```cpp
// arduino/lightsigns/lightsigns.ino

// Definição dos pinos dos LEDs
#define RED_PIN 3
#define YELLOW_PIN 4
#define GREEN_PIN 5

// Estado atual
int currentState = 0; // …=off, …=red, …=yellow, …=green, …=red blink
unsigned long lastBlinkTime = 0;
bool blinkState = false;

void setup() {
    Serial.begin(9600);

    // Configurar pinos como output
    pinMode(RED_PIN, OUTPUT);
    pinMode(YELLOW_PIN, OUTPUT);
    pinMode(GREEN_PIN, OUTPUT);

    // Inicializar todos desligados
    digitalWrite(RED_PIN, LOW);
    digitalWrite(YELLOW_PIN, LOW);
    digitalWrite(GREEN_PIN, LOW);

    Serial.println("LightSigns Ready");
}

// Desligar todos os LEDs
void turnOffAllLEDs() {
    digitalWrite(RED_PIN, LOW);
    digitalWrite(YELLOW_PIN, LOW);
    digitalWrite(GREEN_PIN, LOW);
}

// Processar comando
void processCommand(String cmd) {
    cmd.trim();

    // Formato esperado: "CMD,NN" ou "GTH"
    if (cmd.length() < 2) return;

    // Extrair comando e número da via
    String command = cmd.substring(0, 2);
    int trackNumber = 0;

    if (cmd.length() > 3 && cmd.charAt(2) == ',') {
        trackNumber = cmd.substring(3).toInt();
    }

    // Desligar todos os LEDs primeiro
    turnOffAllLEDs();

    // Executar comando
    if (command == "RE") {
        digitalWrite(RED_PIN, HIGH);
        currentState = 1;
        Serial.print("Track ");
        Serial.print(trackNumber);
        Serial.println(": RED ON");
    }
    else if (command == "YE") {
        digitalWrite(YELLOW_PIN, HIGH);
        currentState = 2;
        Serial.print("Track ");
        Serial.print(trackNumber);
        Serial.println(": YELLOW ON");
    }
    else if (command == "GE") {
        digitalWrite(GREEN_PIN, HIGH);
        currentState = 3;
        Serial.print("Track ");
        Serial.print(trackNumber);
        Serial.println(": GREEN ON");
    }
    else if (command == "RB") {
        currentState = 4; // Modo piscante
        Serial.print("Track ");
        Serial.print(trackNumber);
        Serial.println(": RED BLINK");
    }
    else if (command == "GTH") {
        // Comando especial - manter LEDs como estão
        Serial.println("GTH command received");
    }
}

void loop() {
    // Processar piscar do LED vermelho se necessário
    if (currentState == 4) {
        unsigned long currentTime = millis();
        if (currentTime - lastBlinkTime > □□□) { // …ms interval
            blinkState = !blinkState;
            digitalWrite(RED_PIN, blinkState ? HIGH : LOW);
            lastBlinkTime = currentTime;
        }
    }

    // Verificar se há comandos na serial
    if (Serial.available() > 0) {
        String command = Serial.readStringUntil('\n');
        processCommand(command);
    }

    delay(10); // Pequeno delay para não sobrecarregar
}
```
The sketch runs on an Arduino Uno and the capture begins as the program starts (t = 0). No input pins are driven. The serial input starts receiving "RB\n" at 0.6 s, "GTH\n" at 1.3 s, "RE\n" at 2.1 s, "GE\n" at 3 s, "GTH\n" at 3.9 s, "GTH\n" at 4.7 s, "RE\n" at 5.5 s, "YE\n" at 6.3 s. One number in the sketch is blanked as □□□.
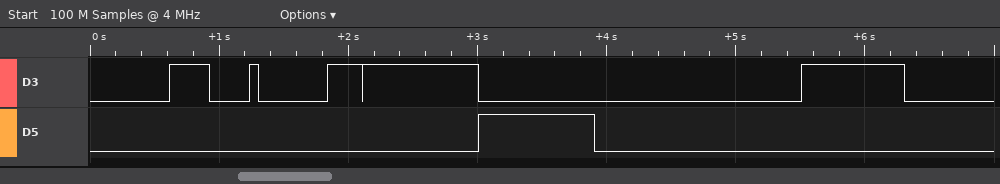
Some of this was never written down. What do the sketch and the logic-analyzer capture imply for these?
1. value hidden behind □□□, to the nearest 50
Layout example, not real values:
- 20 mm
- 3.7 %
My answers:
- 300
